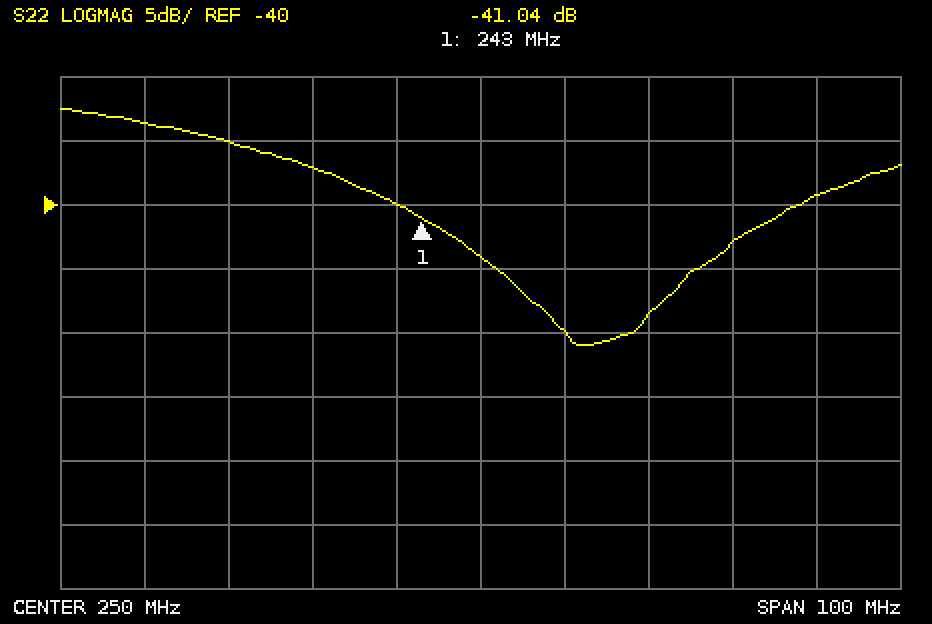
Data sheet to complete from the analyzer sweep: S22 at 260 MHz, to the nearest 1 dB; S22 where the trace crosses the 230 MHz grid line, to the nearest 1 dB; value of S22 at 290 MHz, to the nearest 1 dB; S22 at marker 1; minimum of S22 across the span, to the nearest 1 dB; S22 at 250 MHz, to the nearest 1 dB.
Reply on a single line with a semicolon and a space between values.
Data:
-50 dB; -37 dB; -39 dB; -41.04 dB; -51 dB; -44 dB
